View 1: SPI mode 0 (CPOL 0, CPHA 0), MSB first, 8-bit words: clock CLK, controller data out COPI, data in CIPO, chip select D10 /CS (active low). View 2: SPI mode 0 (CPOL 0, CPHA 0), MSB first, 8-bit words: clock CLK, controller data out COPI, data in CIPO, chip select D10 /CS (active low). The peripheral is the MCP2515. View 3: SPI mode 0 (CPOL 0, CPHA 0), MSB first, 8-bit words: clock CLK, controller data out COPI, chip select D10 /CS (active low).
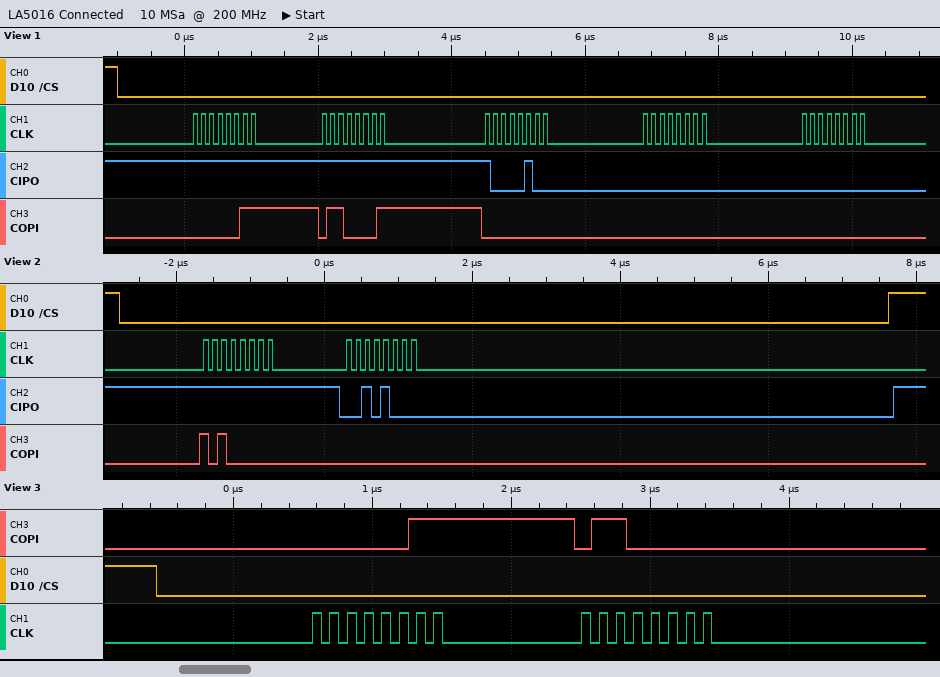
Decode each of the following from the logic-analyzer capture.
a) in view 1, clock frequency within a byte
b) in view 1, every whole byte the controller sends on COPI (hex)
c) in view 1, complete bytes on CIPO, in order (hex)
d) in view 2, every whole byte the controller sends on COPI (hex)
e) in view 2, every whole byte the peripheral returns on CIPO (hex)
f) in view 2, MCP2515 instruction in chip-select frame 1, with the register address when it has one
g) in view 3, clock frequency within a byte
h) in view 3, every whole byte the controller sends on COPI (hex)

8 MHz
03 61 00 00 00
FF FF 84 00 00
A0 00
FF 28
READ STATUS
8 MHz
03 60
